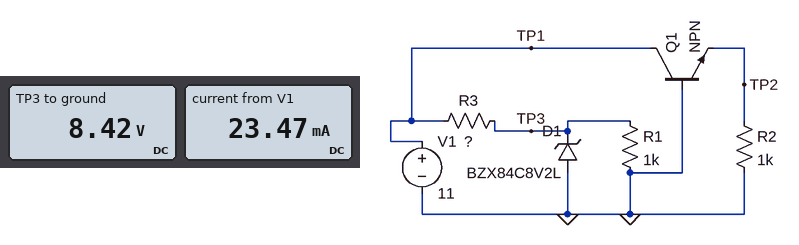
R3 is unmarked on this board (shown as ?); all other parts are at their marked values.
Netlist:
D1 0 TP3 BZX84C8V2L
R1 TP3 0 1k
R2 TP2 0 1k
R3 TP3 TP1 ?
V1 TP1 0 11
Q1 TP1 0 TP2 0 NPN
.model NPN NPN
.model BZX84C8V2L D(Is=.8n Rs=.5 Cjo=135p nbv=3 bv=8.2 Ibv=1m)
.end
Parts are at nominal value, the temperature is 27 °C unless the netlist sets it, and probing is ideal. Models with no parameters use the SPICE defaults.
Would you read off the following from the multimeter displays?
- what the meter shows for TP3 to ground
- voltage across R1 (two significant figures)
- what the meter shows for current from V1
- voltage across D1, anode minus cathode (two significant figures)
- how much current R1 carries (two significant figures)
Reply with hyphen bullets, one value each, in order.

- 8.42 V
- 8.4 V
- 23.47 mA
- -8.4 V
- 8.4 mA
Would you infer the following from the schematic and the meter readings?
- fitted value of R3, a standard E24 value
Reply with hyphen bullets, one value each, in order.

- 110 Ω
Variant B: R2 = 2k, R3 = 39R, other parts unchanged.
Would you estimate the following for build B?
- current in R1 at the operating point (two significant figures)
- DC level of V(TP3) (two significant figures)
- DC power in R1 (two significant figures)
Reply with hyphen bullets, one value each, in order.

- 8.5 mA
- 8.5 V
- 73 mW
